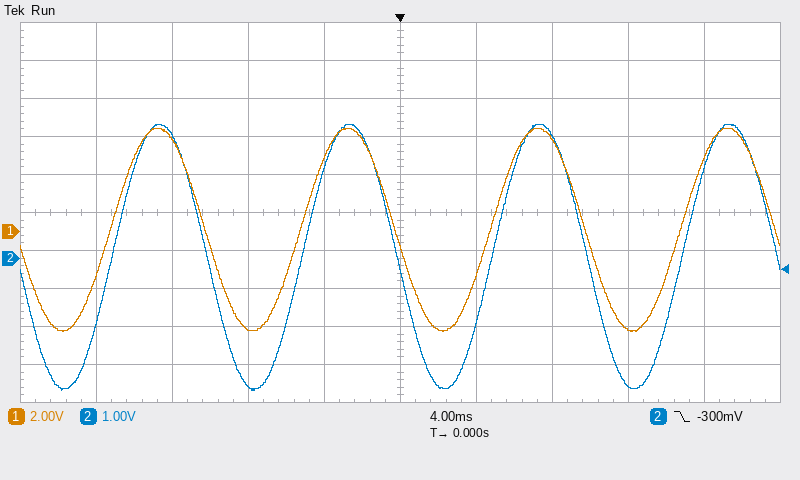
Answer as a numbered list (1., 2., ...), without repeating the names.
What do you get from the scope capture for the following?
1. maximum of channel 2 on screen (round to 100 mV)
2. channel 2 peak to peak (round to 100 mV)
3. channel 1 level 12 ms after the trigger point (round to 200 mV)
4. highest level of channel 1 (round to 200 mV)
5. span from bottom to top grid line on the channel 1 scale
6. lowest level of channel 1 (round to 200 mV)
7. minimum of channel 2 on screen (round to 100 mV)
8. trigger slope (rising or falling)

1. 3.5 V
2. 7.0 V
3. -5.2 V
4. 5.4 V
5. 20 V
6. -5.2 V
7. -3.5 V
8. falling
